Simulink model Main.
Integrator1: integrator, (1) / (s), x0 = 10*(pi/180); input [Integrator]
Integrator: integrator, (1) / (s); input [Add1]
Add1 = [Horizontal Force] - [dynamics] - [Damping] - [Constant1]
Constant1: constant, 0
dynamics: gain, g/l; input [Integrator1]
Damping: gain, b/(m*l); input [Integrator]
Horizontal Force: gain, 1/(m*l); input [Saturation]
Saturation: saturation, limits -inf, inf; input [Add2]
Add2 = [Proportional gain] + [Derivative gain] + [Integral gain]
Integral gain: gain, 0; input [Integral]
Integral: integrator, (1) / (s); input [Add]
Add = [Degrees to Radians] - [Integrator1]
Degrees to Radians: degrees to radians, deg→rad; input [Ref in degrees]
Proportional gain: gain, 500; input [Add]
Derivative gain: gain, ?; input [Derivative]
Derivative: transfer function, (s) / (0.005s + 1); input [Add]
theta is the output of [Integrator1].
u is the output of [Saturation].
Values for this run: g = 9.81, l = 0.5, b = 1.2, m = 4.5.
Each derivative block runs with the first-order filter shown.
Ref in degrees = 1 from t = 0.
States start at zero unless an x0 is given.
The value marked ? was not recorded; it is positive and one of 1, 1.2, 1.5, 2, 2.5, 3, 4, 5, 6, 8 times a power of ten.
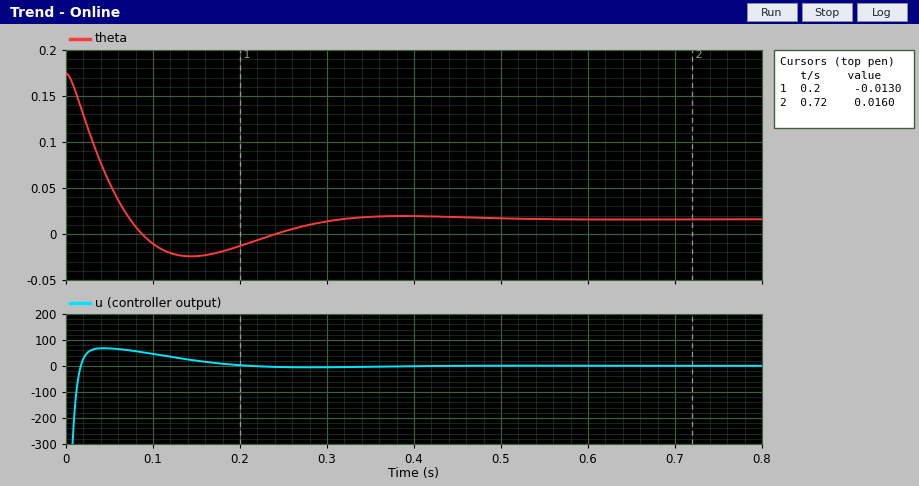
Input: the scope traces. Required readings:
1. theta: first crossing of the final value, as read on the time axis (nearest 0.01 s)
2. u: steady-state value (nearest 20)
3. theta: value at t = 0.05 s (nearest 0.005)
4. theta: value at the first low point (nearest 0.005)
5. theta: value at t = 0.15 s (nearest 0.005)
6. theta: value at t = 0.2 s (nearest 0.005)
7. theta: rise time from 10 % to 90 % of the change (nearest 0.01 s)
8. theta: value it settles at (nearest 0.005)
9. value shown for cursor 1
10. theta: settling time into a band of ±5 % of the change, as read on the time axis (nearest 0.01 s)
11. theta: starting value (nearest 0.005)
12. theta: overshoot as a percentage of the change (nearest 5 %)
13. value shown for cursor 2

0.07 s
0
0.055
-0.025
-0.025
-0.015
0.05 s
0.015
-0.0130
0.27 s
0.175
25 %
0.0160
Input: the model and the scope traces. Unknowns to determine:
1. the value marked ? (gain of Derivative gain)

40
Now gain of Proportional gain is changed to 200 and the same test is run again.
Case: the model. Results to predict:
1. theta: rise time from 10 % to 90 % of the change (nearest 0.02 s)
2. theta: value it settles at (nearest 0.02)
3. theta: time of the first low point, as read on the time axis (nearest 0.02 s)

0.08 s
0.02
0.20 s
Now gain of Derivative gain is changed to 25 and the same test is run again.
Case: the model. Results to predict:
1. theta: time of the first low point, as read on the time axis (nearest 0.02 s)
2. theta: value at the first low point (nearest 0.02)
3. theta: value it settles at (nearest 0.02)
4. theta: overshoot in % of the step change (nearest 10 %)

0.16 s
-0.04
0.02
40 %
